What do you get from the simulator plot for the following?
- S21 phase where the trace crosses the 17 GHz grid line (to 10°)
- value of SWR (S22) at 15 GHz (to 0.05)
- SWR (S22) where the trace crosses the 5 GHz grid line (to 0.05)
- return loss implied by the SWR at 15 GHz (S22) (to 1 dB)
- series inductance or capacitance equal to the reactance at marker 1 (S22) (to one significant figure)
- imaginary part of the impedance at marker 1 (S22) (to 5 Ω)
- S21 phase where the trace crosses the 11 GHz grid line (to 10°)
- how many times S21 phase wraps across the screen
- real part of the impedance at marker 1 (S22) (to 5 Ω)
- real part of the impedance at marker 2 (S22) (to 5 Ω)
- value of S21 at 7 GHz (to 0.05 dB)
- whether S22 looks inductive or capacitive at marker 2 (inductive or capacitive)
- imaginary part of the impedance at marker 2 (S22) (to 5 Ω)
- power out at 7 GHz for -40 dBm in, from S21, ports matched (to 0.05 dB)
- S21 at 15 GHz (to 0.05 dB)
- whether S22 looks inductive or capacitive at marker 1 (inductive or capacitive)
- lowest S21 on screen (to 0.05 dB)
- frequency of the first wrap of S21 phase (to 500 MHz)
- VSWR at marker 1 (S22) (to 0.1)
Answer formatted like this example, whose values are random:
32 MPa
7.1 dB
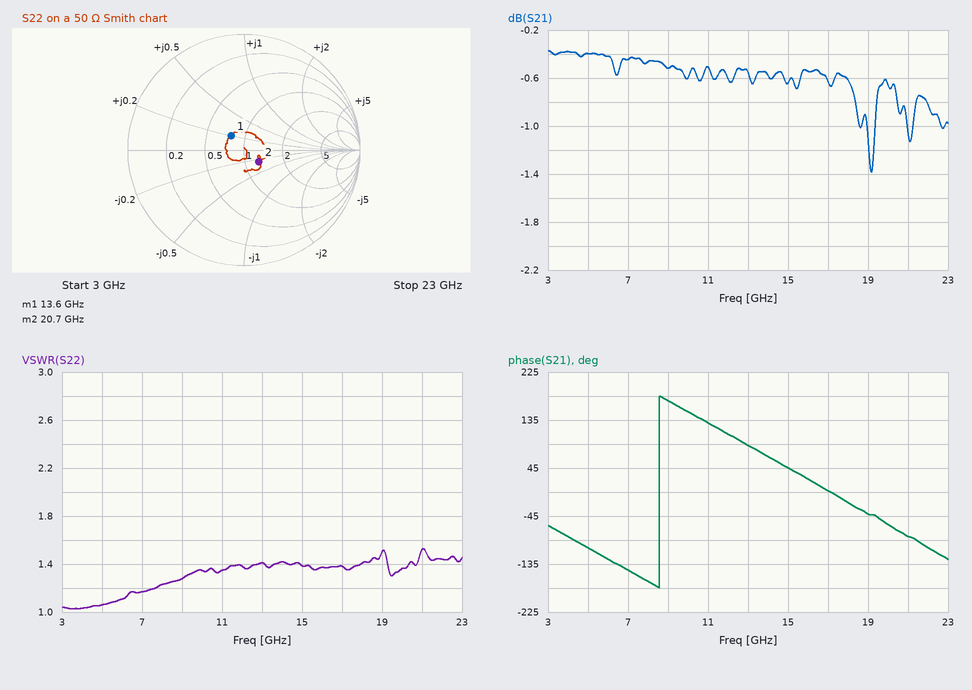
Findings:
0°
1.40
1.05
16 dB
100 pH
+10 Ω
130°
1
40 Ω
65 Ω
-0.45 dB
capacitive
-15 Ω
-40.45 dBm
-0.65 dB
inductive
-1.40 dB
8.5 GHz
1.4
